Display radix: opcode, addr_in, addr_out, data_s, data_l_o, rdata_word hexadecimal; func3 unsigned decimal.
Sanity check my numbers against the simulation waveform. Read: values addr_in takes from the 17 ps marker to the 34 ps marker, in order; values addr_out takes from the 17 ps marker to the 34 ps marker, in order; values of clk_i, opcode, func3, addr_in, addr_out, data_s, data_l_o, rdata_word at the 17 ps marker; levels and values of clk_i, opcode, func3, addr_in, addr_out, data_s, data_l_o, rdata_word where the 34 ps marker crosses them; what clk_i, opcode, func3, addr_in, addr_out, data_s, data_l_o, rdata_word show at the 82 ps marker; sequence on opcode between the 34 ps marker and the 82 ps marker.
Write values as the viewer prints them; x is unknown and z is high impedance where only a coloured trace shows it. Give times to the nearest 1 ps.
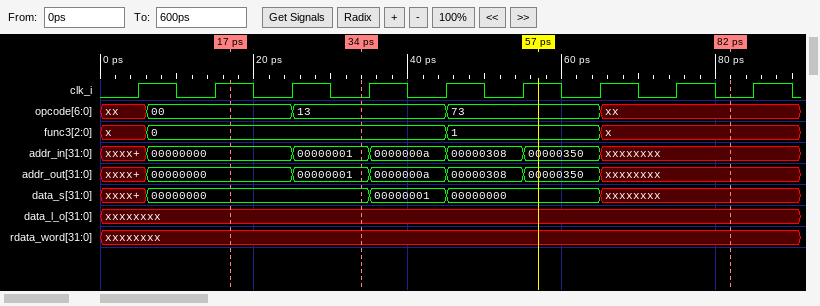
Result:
00000000, 00000001
00000000, 00000001
clk_i=1, opcode=00, func3=0, addr_in=00000000, addr_out=00000000, data_s=00000000, data_l_o=xxxxxxxx, rdata_word=xxxxxxxx
clk_i=0, opcode=13, func3=0, addr_in=00000001, addr_out=00000001, data_s=00000000, data_l_o=xxxxxxxx, rdata_word=xxxxxxxx
clk_i=0, opcode=xx, func3=x, addr_in=xxxxxxxx, addr_out=xxxxxxxx, data_s=xxxxxxxx, data_l_o=xxxxxxxx, rdata_word=xxxxxxxx
13, 73, xx
